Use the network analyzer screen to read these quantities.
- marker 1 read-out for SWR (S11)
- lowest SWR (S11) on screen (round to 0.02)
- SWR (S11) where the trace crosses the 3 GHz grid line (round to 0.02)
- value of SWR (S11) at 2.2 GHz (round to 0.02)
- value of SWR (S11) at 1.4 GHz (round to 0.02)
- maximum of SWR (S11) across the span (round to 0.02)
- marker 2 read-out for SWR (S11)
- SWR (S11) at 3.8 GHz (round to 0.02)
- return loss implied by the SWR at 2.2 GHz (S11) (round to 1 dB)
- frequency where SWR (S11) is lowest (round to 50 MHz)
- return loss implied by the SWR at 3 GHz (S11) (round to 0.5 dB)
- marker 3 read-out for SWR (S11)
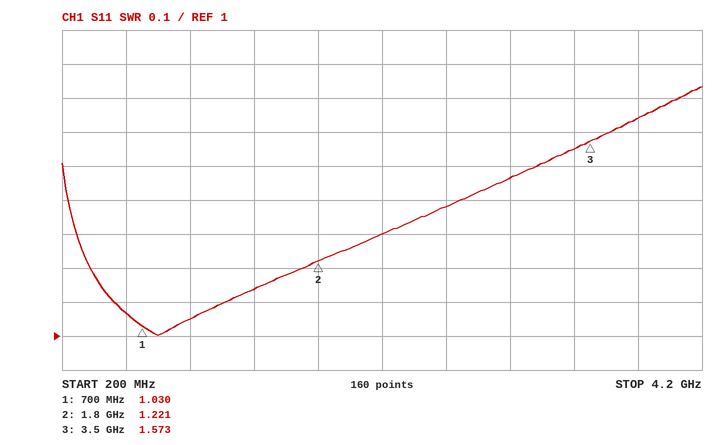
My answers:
1.030
1.00
1.46
1.30
1.14
1.74
1.221
1.64
18 dB
800 MHz
14.5 dB
1.573
